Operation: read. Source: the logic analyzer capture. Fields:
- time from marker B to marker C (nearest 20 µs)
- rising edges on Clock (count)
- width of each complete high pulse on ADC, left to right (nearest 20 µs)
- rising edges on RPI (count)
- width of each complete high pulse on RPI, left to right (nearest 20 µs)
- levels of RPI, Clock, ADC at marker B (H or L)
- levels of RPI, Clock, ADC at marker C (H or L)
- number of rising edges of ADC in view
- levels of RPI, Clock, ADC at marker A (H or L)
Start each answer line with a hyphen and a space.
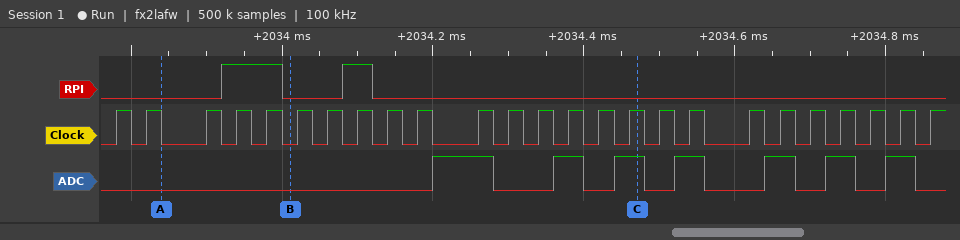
- 460 µs
- 25
- 80 µs, 40 µs, 40 µs, 40 µs, 40 µs, 40 µs, 40 µs
- 2
- 80 µs, 40 µs
- RPI=L, Clock=L, ADC=L
- RPI=L, Clock=H, ADC=H
- 7
- RPI=L, Clock=L, ADC=L
